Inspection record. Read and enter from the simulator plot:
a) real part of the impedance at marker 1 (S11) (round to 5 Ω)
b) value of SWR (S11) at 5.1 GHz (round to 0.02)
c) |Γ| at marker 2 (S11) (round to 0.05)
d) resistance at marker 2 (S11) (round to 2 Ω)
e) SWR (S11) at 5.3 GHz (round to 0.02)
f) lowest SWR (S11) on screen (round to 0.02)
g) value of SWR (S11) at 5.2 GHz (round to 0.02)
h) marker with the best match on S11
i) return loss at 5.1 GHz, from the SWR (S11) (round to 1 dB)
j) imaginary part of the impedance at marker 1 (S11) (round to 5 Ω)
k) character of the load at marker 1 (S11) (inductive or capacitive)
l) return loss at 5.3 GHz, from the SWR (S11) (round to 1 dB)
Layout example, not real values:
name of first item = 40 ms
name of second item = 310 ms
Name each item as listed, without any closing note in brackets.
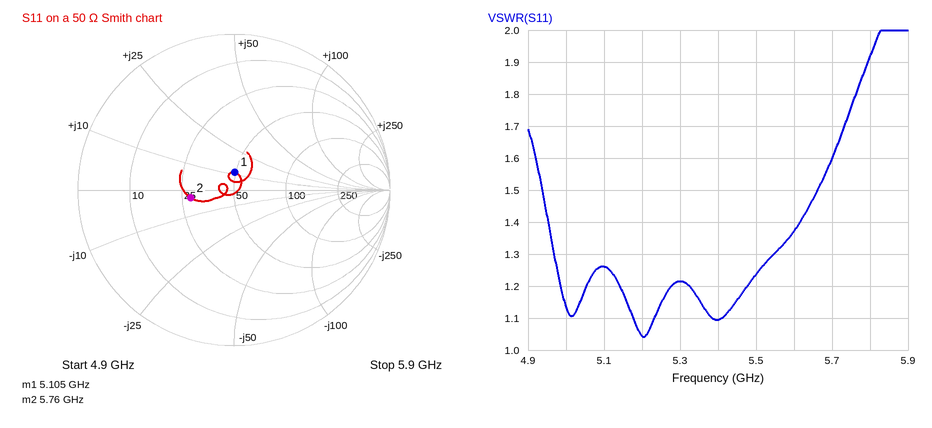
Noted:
real part of the impedance at marker 1 (S11) = 50 Ω
value of SWR (S11) at 5.1 GHz = 1.26
|Γ| at marker 2 (S11) = 0.30
resistance at marker 2 (S11) = 28 Ω
SWR (S11) at 5.3 GHz = 1.22
lowest SWR (S11) on screen = 1.04
value of SWR (S11) at 5.2 GHz = 1.04
marker with the best match on S11 = marker 1
return loss at 5.1 GHz, from the SWR (S11) = 19 dB
imaginary part of the impedance at marker 1 (S11) = +10 Ω
character of the load at marker 1 (S11) = inductive
return loss at 5.3 GHz, from the SWR (S11) = 20 dB
